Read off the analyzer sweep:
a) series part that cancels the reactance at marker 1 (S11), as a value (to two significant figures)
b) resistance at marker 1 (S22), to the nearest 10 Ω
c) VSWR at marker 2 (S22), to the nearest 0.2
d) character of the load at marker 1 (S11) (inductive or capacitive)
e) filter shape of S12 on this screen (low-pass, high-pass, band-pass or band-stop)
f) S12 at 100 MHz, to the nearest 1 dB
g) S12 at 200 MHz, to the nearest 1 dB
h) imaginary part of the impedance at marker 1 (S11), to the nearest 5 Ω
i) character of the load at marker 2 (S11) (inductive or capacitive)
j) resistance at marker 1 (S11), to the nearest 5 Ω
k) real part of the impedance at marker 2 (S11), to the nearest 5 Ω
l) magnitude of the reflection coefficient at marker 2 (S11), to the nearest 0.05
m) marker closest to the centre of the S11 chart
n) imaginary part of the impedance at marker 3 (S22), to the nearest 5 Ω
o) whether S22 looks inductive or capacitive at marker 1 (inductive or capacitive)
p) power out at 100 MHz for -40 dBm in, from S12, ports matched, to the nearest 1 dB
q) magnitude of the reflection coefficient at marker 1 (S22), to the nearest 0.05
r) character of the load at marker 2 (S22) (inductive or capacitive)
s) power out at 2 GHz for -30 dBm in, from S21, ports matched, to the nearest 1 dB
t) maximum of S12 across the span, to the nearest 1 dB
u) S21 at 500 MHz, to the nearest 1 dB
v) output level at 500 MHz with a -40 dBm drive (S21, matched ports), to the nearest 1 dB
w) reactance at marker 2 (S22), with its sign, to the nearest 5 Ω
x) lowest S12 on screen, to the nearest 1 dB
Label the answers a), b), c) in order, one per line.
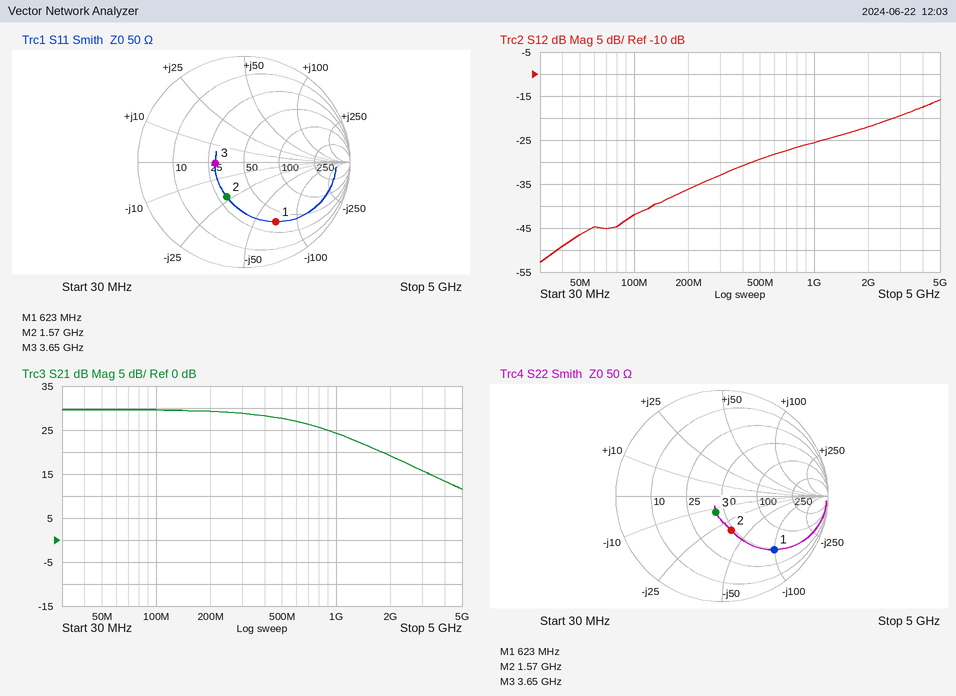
a) 18 nH
b) 50 Ω
c) 2.0
d) capacitive
e) high-pass
f) -42 dB
g) -36 dB
h) -70 Ω
i) capacitive
j) 35 Ω
k) 30 Ω
l) 0.35
m) marker 3
n) -15 Ω
o) capacitive
p) -82 dBm
q) 0.70
r) capacitive
s) -11 dBm
t) -16 dB
u) 28 dB
v) -12 dBm
w) -35 Ω
x) -53 dB
